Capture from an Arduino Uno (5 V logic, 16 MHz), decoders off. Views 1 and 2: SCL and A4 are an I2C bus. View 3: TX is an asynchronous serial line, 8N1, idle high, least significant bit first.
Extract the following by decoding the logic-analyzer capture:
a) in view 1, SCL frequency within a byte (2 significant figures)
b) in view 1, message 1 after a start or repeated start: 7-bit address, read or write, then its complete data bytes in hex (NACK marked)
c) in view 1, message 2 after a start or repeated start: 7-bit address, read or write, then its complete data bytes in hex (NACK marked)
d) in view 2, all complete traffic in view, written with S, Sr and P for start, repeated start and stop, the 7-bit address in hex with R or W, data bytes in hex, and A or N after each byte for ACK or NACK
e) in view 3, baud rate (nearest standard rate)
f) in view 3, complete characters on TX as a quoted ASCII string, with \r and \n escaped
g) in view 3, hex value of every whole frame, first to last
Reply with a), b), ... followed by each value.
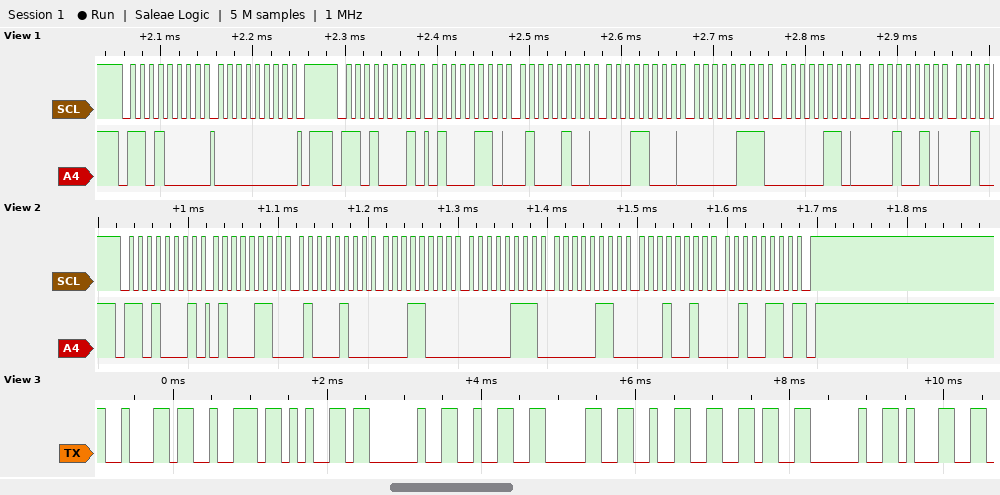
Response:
a) 100 kHz
b) 0x68 write: 00
c) 0x68 read: 46 44 18 07 06 12
d) S 68R A 46 A 44 A 18 A 07 A 06 A 12 A 26 N P
e) 9600 baud
f) "bre 2026 1"
g) 62 72 65 20 32 30 32 36 20 31
